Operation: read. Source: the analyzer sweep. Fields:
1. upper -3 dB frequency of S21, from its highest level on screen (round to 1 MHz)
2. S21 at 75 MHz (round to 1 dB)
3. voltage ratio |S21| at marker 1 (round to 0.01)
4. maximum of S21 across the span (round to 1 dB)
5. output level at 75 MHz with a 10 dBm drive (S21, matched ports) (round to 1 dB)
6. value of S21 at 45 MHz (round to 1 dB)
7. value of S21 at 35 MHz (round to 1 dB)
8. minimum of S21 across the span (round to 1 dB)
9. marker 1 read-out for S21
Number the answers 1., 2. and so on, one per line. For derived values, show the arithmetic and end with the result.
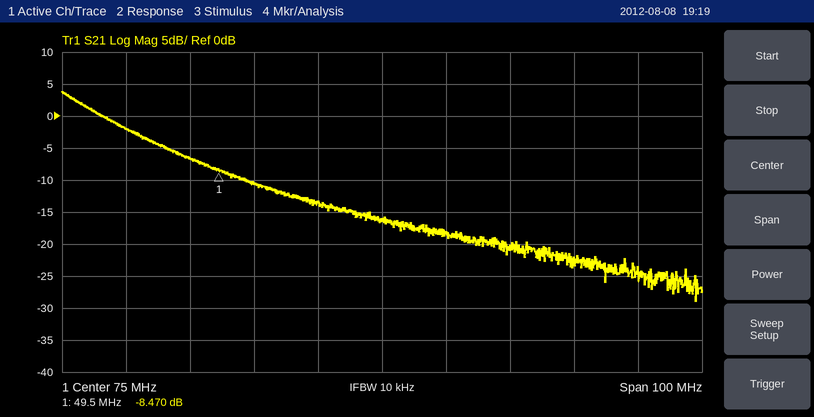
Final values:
1. 30 MHz
2. -16 dB
3. 10^(-8.47/20) ≈ 0.38
4. 4 dB
5. 10 dBm + (-16 dB) = -6 dBm
6. -7 dB
7. -2 dB
8. -29 dB
9. -8.470 dB
